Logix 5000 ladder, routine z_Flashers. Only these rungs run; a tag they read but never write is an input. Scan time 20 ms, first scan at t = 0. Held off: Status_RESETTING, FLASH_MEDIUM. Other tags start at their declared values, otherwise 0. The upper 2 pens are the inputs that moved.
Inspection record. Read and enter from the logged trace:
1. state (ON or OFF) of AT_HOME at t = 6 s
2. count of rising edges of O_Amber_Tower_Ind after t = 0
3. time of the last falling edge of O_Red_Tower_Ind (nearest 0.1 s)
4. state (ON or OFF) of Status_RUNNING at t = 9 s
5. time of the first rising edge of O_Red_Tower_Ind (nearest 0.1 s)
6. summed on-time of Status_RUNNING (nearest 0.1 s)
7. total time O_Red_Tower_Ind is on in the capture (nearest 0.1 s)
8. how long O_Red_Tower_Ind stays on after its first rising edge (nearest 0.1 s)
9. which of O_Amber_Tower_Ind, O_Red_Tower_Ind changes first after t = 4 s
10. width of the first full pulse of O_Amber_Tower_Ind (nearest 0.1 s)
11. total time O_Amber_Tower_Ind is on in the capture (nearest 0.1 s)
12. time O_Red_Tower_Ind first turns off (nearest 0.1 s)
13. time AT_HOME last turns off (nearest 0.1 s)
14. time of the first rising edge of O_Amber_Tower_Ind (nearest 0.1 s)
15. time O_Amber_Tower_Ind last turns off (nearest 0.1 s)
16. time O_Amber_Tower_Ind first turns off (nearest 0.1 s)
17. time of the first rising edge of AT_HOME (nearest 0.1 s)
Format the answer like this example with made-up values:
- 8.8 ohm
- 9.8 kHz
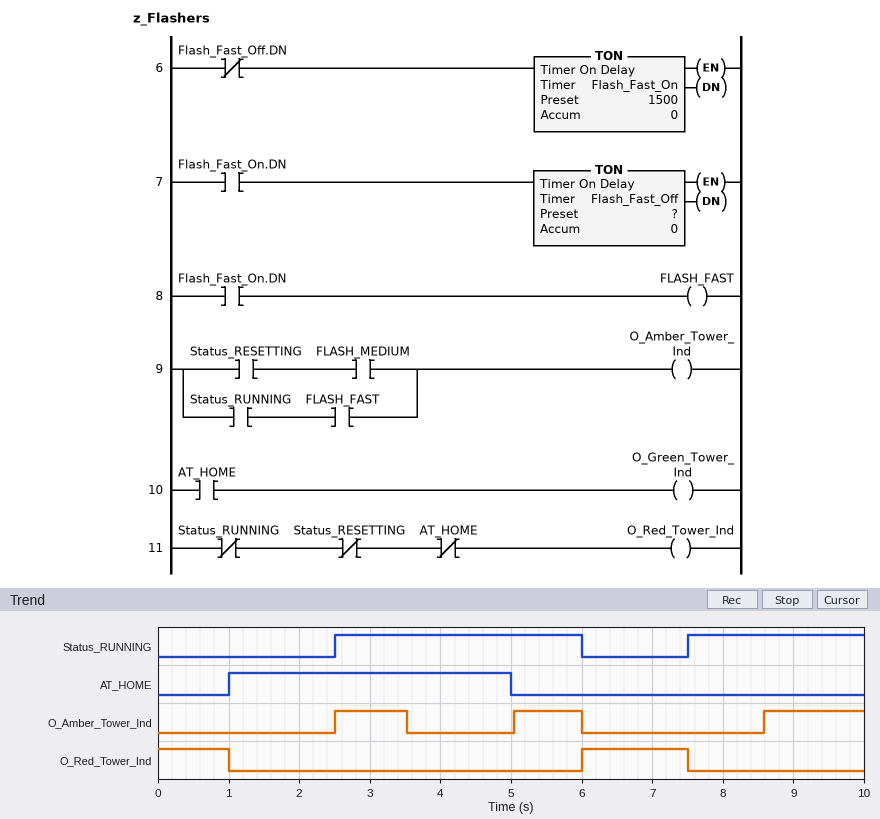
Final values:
- OFF
- 3
- 7.5 s
- ON
- 6.0 s
- 6.0 s
- 2.5 s
- 1.5 s
- O_Amber_Tower_Ind
- 1.0 s
- 3.4 s
- 1.0 s
- 5.0 s
- 2.5 s
- 6.0 s
- 3.5 s
- 1.0 s
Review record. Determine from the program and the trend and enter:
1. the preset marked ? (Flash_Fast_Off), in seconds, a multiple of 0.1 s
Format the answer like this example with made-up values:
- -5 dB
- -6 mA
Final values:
- 2.0 s
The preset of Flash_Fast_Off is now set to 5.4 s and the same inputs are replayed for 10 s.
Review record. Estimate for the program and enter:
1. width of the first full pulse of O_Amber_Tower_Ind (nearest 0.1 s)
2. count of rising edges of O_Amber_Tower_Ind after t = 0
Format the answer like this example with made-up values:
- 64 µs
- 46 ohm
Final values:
- 3.5 s
- 2
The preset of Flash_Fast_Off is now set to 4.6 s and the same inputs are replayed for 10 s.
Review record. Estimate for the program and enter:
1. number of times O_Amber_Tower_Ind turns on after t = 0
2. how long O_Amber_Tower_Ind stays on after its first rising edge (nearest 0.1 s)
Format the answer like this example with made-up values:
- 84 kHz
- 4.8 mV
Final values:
- 2
- 3.5 s
